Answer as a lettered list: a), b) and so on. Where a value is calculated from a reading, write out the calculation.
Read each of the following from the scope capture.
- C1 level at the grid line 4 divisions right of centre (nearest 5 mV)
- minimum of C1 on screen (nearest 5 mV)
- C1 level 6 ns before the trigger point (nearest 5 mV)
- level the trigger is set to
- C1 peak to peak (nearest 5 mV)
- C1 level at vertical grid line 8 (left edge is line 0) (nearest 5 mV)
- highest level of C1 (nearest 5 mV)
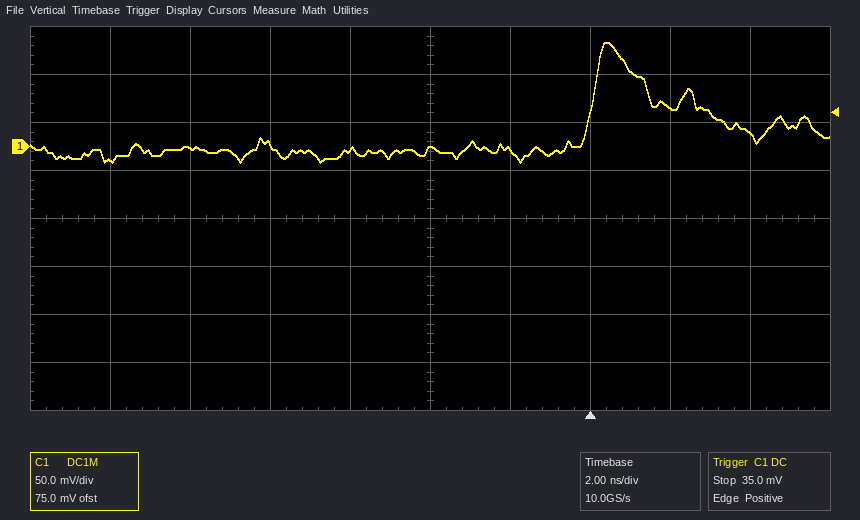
a) 15 mV
b) -15 mV
c) -5 mV
d) 35.0 mV
e) 110 mV − (-15 mV) = 125 mV
f) 40 mV
g) 110 mV
